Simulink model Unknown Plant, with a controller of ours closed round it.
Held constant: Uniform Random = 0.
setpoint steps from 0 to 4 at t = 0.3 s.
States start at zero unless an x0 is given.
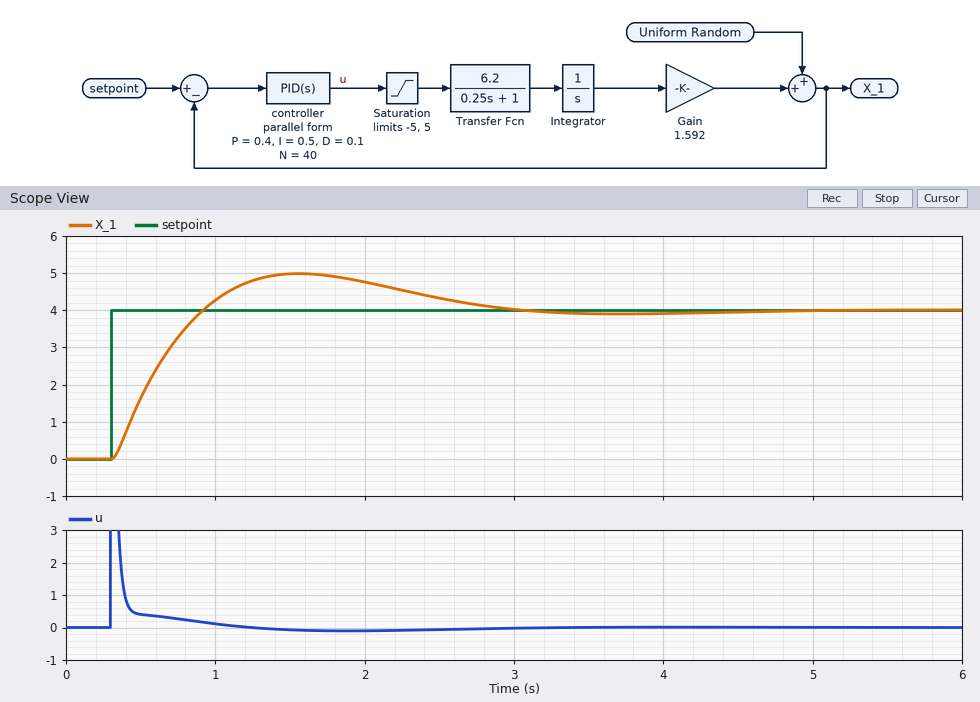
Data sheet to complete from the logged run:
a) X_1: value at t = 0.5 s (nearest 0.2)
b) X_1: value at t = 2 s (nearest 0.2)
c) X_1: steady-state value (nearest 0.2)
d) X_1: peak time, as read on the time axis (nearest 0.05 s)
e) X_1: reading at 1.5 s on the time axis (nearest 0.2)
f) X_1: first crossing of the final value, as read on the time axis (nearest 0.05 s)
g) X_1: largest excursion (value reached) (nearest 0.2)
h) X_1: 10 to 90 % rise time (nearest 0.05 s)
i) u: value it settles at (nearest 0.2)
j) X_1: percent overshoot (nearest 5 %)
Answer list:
1.6
4.8
4.0
1.55 s
5.0
0.90 s
5.0
0.45 s
0.0
25 %
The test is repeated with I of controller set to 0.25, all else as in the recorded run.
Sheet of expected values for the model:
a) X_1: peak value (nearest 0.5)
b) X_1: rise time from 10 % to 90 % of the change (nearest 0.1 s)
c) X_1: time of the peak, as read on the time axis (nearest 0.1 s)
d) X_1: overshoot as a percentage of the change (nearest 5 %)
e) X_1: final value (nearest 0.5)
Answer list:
4.5
0.5 s
1.8 s
15 %
4.0
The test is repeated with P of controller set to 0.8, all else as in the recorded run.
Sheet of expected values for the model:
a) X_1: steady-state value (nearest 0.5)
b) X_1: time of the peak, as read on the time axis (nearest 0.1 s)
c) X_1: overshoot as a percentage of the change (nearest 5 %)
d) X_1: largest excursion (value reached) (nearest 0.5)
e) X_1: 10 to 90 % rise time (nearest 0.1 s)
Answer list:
4.0
1.0 s
15 %
4.5
0.3 s
